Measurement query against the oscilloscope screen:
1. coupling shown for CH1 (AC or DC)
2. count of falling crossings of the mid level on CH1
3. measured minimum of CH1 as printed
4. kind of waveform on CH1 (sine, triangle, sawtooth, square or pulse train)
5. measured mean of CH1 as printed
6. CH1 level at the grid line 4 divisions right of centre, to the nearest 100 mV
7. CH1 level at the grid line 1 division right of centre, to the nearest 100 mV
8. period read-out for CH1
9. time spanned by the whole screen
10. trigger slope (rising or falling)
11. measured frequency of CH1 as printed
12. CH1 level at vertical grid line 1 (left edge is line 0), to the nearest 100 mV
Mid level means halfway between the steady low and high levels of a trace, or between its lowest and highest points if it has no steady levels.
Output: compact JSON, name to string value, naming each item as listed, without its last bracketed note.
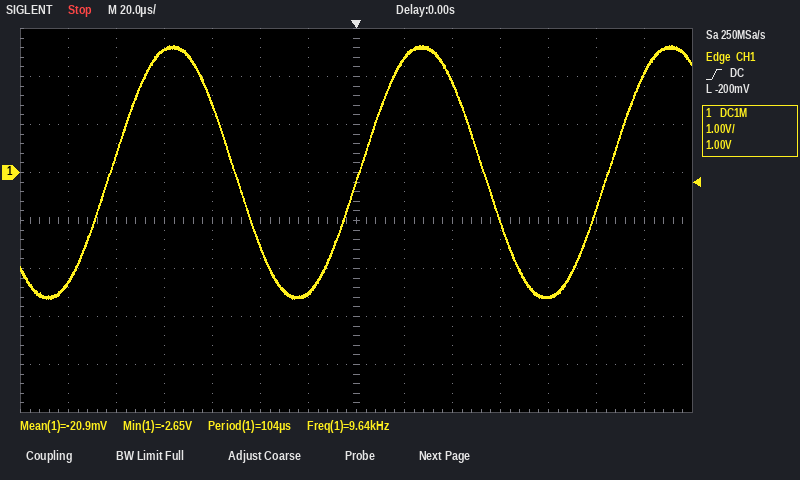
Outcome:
{"coupling shown for CH1": "DC", "count of falling crossings of the mid level on CH1": "2", "measured minimum of CH1 as printed": "-2.65 V", "kind of waveform on CH1": "sine", "measured mean of CH1 as printed": "-20.9 mV", "CH1 level at the grid line 4 divisions right of centre, to the nearest 100 mV": "-2.6 V", "CH1 level at the grid line 1 division right of centre, to the nearest 100 mV": "2.4 V", "period read-out for CH1": "104 µs", "time spanned by the whole screen": "280 µs", "trigger slope": "rising", "measured frequency of CH1 as printed": "9.64 kHz", "CH1 level at vertical grid line 1 (left edge is line 0), to the nearest 100 mV": "-2.3 V"}
